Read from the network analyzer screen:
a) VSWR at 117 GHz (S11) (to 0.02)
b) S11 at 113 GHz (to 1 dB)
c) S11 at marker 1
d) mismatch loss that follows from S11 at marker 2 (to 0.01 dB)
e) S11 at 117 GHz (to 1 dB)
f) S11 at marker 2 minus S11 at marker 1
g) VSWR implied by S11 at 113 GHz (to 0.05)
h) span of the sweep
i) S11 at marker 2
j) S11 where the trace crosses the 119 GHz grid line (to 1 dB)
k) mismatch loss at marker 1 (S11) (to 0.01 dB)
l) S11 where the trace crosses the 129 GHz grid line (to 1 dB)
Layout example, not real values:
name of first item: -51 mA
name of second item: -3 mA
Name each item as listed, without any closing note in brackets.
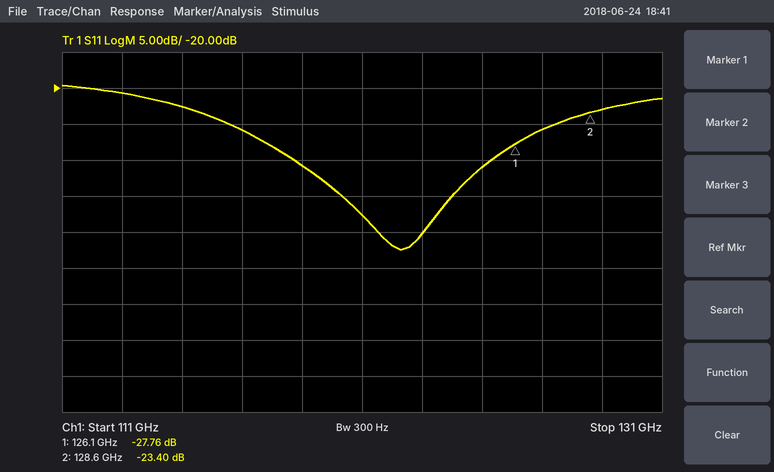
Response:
VSWR at 117 GHz (S11): 1.10
S11 at 113 GHz: -21 dB
S11 at marker 1: -27.76 dB
mismatch loss that follows from S11 at marker 2: 0.02 dB
S11 at 117 GHz: -26 dB
S11 at marker 2 minus S11 at marker 1: 4.36 dB
VSWR implied by S11 at 113 GHz: 1.20
span of the sweep: 20 GHz
S11 at marker 2: -23.40 dB
S11 where the trace crosses the 119 GHz grid line: -31 dB
mismatch loss at marker 1 (S11): 0.01 dB
S11 where the trace crosses the 129 GHz grid line: -23 dB
